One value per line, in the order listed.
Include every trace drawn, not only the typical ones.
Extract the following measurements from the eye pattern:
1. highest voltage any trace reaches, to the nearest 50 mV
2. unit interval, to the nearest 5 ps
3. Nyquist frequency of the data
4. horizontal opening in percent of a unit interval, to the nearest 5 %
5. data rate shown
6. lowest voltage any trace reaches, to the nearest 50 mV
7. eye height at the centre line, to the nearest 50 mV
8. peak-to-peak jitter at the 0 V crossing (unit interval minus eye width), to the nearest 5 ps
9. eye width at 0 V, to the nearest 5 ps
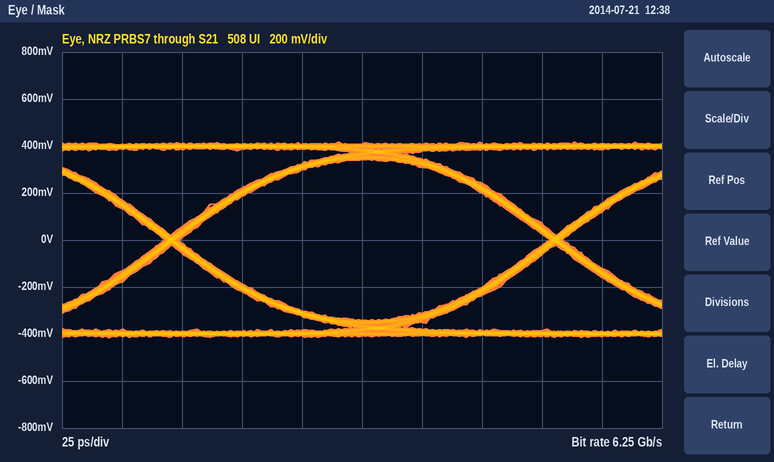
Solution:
400 mV
160 ps
3.125 GHz
95 %
6.25 Gb/s
-400 mV
700 mV
5 ps
155 ps
